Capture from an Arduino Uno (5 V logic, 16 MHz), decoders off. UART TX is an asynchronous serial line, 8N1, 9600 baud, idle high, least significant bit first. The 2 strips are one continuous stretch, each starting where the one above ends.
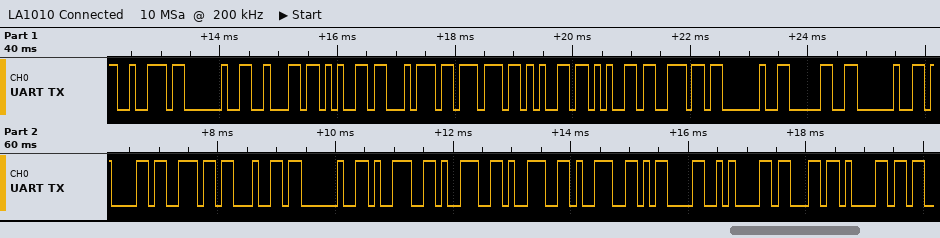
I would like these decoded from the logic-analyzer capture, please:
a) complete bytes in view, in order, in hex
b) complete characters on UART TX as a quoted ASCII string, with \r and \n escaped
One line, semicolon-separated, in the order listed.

72 20 62 65 74 77 65 65 6E 20 30 20 61 6E 64 20 39 39 39 39 0D 0A 63 61; "r between 0 and 9999\r\nca"
